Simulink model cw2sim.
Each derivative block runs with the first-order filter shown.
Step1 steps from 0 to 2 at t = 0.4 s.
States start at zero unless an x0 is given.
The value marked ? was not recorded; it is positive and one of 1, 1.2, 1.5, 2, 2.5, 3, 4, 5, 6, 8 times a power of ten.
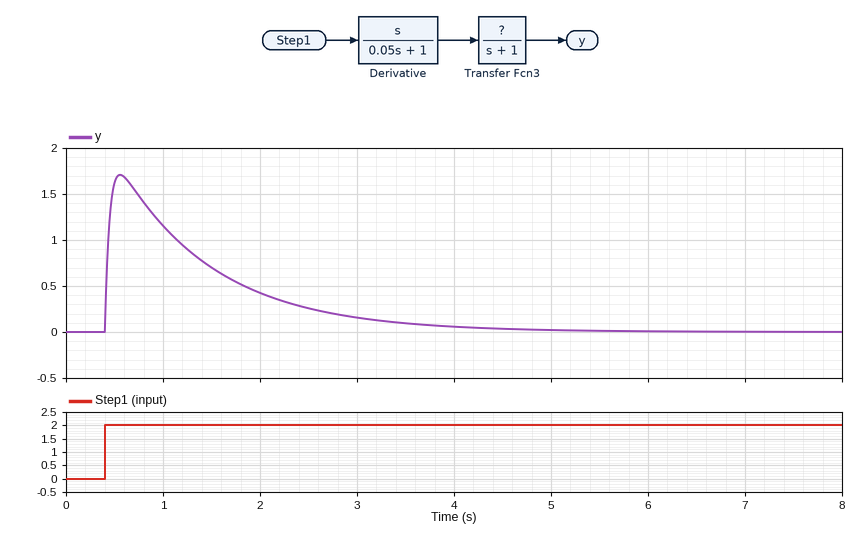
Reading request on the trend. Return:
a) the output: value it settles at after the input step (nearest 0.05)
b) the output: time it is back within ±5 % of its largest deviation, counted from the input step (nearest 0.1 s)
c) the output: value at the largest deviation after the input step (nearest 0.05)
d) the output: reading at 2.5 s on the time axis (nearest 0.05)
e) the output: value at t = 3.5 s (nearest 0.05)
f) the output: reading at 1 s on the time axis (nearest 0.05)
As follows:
0.00
3.2 s
1.70
0.25
0.10
1.15
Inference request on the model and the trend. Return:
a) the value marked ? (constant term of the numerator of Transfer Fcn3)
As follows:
1
